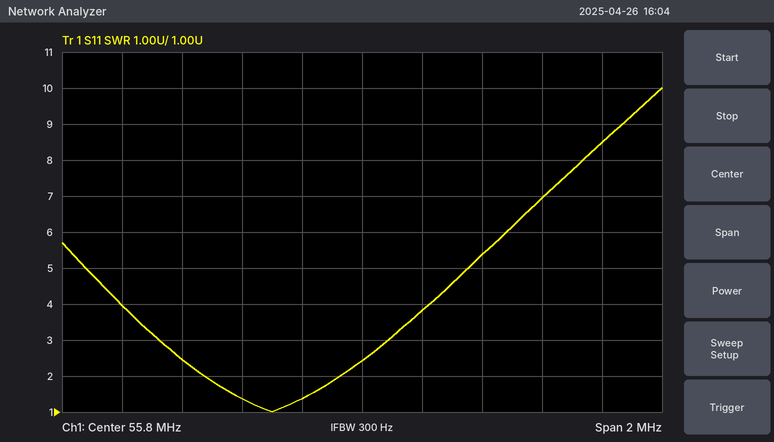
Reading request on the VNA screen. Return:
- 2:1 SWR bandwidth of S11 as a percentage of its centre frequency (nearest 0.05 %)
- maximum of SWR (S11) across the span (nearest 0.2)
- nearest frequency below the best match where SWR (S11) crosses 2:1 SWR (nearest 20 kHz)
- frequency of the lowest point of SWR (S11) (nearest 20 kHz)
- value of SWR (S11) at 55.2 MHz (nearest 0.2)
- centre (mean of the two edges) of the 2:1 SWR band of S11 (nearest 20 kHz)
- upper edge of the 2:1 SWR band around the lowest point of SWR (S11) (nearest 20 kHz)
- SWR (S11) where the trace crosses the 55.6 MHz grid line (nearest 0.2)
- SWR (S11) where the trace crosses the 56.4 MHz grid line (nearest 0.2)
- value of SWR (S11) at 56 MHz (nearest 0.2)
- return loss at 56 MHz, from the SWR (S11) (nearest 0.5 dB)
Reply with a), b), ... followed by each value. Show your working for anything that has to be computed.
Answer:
a) 440 kHz / 55.5 MHz ≈ 0.793 %, so 0.80 % to the nearest 0.05 %
b) 10.0
c) 55.28 MHz
d) 55.50 MHz
e) 2.4
f) 55.50 MHz
g) 55.72 MHz
h) 1.4
i) 7.0
j) 3.8
k) −20 log10((3.8 − 1)/(3.8 + 1)) ≈ 4.68 dB, so 4.5 dB to the nearest 0.5 dB
